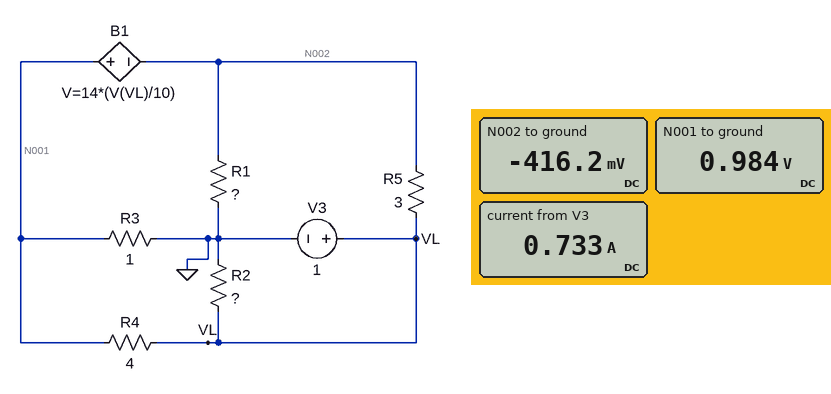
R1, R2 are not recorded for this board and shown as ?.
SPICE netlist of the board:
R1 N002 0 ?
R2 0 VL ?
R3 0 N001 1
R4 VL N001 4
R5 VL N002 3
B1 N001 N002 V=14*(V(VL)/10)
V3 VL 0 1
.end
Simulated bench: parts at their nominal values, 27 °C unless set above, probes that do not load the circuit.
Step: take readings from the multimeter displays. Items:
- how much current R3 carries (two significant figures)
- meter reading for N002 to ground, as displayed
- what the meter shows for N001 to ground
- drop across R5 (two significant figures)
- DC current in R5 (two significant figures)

980 mA
-416.2 mV
0.984 V
1.4 V
470 mA
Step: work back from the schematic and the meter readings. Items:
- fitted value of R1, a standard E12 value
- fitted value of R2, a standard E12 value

0.82 Ω
3.9 Ω
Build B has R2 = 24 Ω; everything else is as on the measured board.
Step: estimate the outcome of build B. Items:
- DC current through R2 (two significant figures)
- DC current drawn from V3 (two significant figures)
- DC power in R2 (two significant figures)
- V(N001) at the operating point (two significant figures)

42 mA
520 mA
42 mW
980 mV
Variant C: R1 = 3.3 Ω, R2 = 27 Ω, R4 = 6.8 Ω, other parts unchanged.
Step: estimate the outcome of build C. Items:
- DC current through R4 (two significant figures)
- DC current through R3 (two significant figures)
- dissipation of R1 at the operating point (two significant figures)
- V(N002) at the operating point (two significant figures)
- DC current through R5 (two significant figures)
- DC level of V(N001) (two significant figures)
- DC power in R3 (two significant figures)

34 mA
770 mA
120 mW
-630 mV
540 mA
770 mV
590 mW
